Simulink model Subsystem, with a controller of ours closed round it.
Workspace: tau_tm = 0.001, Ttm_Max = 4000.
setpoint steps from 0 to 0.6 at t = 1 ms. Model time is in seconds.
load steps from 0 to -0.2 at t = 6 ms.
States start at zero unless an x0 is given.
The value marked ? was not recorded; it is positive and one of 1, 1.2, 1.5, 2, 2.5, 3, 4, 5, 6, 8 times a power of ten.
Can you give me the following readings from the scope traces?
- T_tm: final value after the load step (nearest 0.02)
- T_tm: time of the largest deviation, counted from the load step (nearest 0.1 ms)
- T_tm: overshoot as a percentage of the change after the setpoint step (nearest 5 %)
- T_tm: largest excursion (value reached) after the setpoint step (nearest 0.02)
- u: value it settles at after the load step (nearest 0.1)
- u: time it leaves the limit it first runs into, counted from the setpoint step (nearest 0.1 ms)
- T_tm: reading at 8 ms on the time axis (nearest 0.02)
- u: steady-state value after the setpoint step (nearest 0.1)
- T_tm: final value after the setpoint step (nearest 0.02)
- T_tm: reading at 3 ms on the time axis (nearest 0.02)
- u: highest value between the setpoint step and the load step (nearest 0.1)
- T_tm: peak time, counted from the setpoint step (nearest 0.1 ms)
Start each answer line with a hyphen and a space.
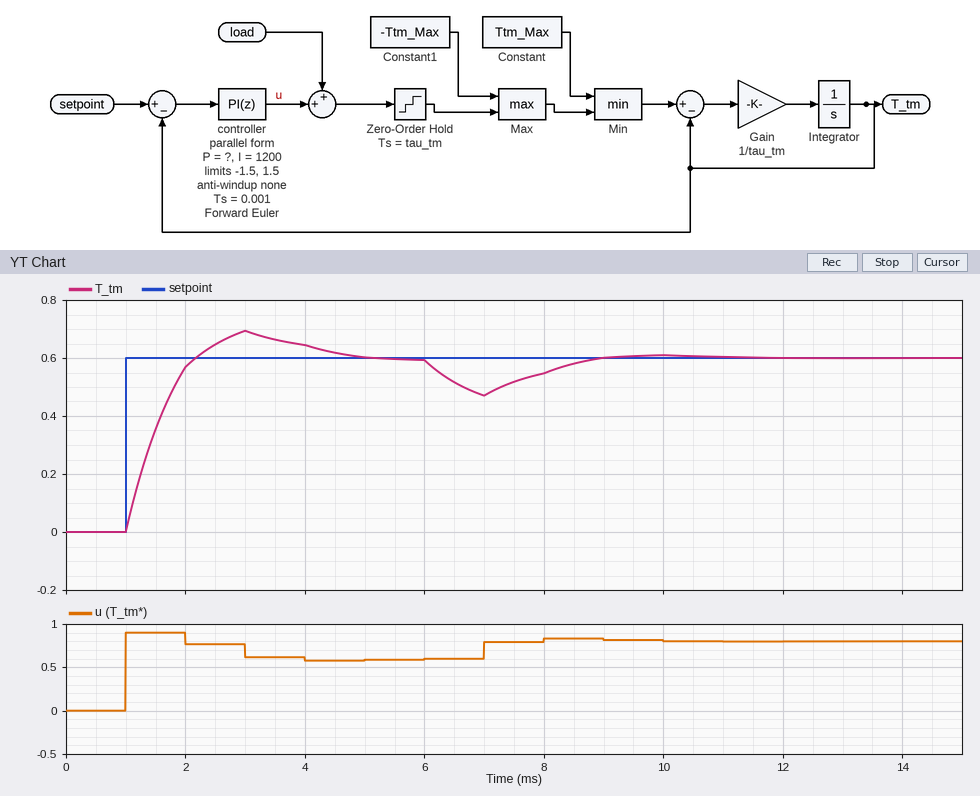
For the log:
- 0.60
- 1.0 ms
- 15 %
- 0.70
- 0.8
- 1.0 ms
- 0.54
- 0.6
- 0.60
- 0.70
- 0.9
- 2.0 ms
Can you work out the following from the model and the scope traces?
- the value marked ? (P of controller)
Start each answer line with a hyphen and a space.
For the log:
- 1.5
